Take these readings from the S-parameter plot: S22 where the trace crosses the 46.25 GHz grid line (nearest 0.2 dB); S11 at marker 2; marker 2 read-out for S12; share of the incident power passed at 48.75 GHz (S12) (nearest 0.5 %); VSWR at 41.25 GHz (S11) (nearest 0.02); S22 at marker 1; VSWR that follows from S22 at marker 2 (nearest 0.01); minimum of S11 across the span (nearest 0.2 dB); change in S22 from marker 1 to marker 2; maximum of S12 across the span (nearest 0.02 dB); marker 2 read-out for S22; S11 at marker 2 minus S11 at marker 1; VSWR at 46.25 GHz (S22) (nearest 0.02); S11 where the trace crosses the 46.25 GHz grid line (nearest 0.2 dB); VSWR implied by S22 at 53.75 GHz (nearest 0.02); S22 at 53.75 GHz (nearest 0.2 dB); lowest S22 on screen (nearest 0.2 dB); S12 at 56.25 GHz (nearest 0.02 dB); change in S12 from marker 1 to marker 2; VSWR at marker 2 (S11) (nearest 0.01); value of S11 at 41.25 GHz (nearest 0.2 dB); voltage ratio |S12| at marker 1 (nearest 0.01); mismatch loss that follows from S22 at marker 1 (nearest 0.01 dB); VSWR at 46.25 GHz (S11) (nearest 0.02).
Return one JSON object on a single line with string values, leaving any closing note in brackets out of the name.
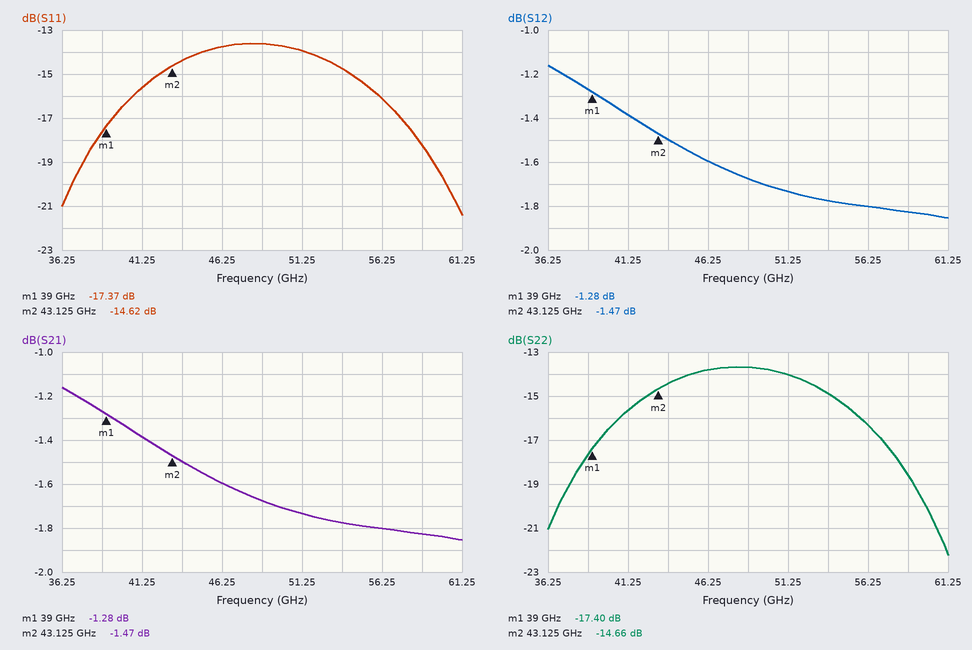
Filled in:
{"S22 where the trace crosses the 46.25 GHz grid line": "-13.8 dB", "S11 at marker 2": "-14.62 dB", "marker 2 read-out for S12": "-1.47 dB", "share of the incident power passed at 48.75 GHz (S12)": "68.0 %", "VSWR at 41.25 GHz (S11)": "1.40", "S22 at marker 1": "-17.40 dB", "VSWR that follows from S22 at marker 2": "1.45", "minimum of S11 across the span": "-21.4 dB", "change in S22 from marker 1 to marker 2": "2.74 dB", "maximum of S12 across the span": "-1.16 dB", "marker 2 read-out for S22": "-14.66 dB", "S11 at marker 2 minus S11 at marker 1": "2.75 dB", "VSWR at 46.25 GHz (S22)": "1.52", "S11 where the trace crosses the 46.25 GHz grid line": "-13.8 dB", "VSWR implied by S22 at 53.75 GHz": "1.44", "S22 at 53.75 GHz": "-14.8 dB", "lowest S22 on screen": "-22.2 dB", "S12 at 56.25 GHz": "-1.80 dB", "change in S12 from marker 1 to marker 2": "-0.19 dB", "VSWR at marker 2 (S11)": "1.46", "value of S11 at 41.25 GHz": "-15.6 dB", "voltage ratio |S12| at marker 1": "0.86", "mismatch loss that follows from S22 at marker 1": "0.08 dB", "VSWR at 46.25 GHz (S11)": "1.52"}
